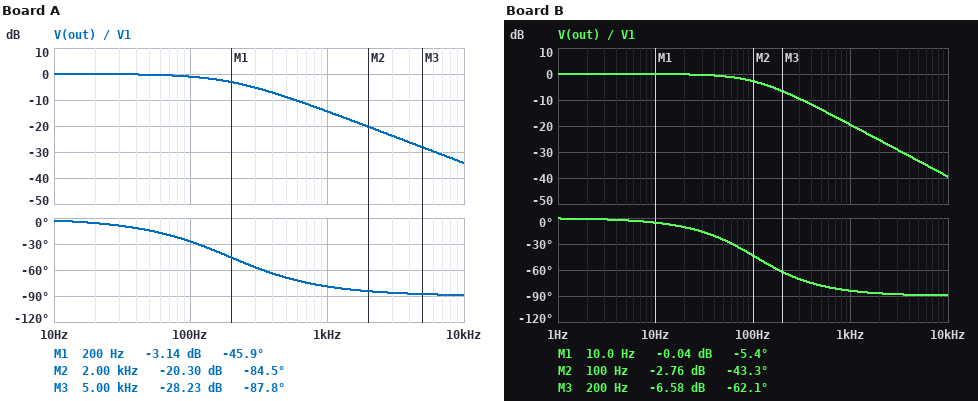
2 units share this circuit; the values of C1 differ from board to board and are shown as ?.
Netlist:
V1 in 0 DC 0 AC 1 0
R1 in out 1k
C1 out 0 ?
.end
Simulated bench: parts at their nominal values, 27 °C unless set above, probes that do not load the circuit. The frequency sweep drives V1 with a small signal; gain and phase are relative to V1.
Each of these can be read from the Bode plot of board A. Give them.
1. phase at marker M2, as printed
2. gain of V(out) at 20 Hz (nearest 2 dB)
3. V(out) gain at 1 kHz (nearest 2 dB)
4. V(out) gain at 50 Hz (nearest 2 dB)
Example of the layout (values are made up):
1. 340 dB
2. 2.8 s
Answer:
1. -84.5 deg
2. 0 dB
3. -14 dB
4. 0 dB
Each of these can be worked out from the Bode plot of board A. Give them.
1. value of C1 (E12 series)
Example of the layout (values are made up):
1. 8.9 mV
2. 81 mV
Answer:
1. 820 nF
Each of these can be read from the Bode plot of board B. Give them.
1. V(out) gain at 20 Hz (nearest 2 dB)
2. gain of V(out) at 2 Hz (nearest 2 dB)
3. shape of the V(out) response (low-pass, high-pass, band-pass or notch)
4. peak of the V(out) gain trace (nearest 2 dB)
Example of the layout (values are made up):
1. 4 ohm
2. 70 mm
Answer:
1. 0 dB
2. 0 dB
3. low-pass
4. 0 dB
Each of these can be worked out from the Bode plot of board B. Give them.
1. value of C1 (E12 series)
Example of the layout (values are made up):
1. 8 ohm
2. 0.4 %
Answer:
1. 1.5 µF
